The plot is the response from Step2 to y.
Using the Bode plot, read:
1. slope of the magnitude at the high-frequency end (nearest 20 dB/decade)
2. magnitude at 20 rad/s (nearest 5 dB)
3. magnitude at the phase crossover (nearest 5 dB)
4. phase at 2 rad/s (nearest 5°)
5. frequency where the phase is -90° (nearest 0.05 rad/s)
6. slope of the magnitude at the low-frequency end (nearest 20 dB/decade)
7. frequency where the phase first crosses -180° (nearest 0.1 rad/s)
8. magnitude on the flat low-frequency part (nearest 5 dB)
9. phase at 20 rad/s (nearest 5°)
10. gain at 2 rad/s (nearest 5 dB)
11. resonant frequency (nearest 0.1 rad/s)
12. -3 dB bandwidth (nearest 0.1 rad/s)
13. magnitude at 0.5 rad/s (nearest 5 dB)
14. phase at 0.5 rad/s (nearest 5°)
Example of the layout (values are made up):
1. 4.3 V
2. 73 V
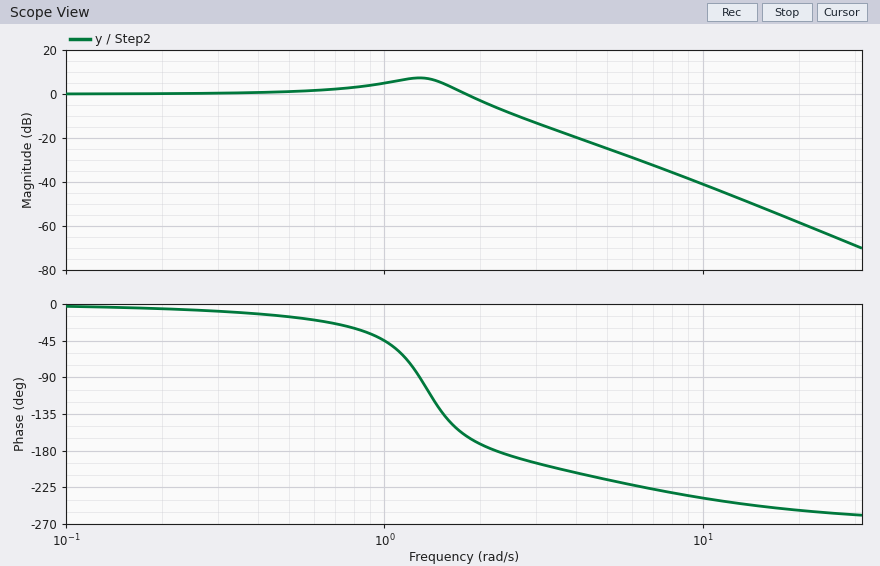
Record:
1. -60 dB/decade
2. -60 dB
3. -5 dB
4. -170°
5. 1.30 rad/s
6. 0 dB/decade
7. 2.2 rad/s
8. 0 dB
9. -255°
10. -5 dB
11. 1.3 rad/s
12. 2.0 rad/s
13. 0 dB
14. -15°
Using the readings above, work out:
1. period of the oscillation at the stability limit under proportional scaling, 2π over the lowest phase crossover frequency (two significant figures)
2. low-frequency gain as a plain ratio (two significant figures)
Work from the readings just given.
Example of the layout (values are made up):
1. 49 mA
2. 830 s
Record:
1. 2.9 s
2. 1.0
